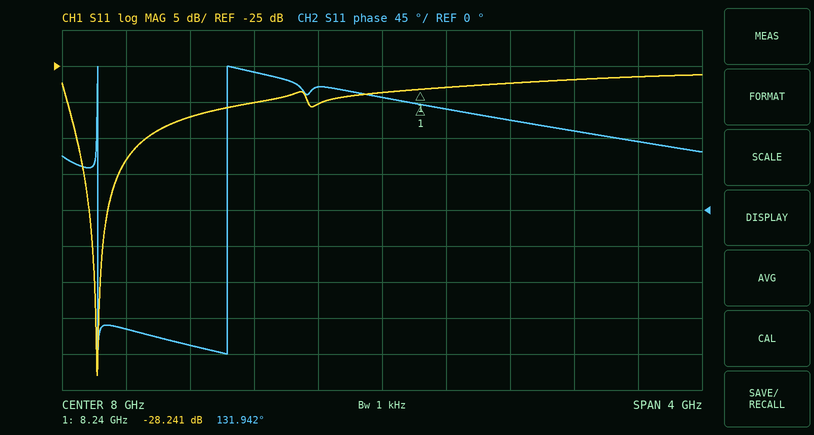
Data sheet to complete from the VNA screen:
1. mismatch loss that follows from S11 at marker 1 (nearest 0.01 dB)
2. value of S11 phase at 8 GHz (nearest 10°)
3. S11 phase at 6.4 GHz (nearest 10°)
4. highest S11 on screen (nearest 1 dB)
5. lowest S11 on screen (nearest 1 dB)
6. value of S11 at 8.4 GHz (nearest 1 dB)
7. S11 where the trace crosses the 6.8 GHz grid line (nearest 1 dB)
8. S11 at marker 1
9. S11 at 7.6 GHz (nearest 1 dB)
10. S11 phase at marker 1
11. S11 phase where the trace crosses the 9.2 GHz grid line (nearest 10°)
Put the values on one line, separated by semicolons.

0.01 dB; 140°; -150°; -26 dB; -68 dB; -28 dB; -32 dB; -28.241 dB; -30 dB; 131.942°; 100°
